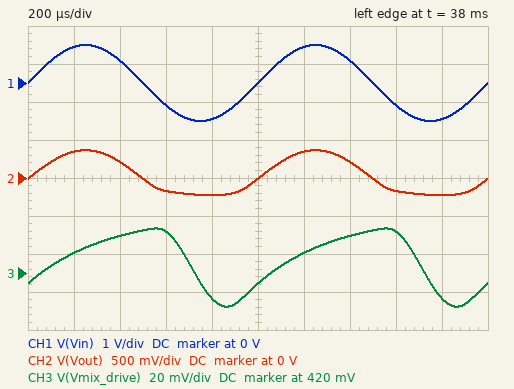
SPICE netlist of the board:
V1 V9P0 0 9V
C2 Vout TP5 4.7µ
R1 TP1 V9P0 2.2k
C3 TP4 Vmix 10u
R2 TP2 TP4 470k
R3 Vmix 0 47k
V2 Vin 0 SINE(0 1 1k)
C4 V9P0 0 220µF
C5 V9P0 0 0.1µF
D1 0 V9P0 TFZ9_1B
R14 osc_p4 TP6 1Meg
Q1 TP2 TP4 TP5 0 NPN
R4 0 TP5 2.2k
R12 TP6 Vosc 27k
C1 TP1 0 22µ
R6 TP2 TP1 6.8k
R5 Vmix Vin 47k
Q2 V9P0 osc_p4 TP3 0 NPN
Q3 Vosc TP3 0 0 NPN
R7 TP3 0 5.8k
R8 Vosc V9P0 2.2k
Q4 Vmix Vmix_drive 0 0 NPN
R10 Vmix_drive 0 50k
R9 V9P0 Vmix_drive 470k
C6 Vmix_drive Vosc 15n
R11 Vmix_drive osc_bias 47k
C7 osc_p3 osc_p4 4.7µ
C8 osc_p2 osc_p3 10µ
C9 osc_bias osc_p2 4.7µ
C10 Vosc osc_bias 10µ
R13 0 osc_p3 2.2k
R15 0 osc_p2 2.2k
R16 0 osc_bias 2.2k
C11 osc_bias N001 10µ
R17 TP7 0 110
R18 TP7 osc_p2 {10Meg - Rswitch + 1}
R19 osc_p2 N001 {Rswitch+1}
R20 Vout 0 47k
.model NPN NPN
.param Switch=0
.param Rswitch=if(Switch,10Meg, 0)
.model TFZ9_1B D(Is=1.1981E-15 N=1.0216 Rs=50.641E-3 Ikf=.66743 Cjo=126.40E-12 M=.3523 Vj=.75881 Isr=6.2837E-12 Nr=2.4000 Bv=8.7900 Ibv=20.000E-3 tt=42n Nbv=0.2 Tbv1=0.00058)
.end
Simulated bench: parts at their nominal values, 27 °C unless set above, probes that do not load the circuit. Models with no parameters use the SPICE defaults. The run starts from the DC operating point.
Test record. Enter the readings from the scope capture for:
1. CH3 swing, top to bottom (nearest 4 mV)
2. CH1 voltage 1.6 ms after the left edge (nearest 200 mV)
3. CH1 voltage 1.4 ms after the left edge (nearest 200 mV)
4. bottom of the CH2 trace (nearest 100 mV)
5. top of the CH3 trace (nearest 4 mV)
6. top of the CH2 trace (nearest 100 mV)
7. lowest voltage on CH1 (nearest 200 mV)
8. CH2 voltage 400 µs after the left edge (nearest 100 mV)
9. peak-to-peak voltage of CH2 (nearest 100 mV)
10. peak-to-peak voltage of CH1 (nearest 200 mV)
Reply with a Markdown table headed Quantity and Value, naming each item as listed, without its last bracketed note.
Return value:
| Quantity | Value |
|---|---|
| CH3 swing, top to bottom | 40 mV |
| CH1 voltage 1.6 ms after the left edge | -600 mV |
| CH1 voltage 1.4 ms after the left edge | 600 mV |
| bottom of the CH2 trace | -200 mV |
| top of the CH3 trace | 444 mV |
| top of the CH2 trace | 400 mV |
| lowest voltage on CH1 | -1.0 V |
| CH2 voltage 400 µs after the left edge | 200 mV |
| peak-to-peak voltage of CH2 | 600 mV |
| peak-to-peak voltage of CH1 | 2.0 V |
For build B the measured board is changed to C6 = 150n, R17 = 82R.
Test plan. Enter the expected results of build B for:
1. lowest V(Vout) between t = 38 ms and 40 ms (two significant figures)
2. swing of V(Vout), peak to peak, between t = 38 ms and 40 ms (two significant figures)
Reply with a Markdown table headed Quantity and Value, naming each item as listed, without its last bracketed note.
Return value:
| Quantity | Value |
|---|---|
| lowest V(Vout) between t = 38 ms and 40 ms | -210 mV |
| swing of V(Vout), peak to peak, between t = 38 ms and 40 ms | 580 mV |
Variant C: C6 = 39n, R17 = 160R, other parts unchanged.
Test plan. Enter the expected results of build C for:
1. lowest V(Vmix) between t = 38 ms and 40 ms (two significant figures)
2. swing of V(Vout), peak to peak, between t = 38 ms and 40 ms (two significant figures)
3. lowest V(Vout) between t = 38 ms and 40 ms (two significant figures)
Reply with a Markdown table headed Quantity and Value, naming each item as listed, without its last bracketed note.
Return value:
| Quantity | Value |
|---|---|
| lowest V(Vmix) between t = 38 ms and 40 ms | -210 mV |
| swing of V(Vout), peak to peak, between t = 38 ms and 40 ms | 580 mV |
| lowest V(Vout) between t = 38 ms and 40 ms | -220 mV |
